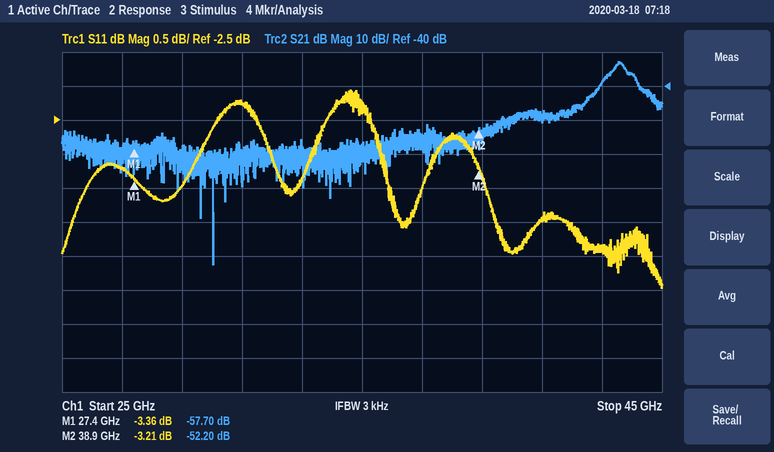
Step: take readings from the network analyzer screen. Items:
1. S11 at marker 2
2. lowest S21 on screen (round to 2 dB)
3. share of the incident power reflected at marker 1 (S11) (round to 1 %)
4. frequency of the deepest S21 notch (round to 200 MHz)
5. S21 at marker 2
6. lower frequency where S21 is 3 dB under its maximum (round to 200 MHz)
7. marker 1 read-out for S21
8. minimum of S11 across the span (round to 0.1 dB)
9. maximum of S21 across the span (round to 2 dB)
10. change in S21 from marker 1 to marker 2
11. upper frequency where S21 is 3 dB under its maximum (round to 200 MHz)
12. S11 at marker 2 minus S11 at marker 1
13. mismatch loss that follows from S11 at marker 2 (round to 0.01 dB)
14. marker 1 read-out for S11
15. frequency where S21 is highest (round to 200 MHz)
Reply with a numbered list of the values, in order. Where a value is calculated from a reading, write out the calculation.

1. -3.21 dB
2. -92 dB
3. 10^(-3.36/10) ≈ 46 %
4. 30.0 GHz
5. -52.20 dB
6. 43.4 GHz
7. -57.70 dB
8. -5.0 dB
9. -32 dB
10. -52.2 − (-57.7) = 5.50 dB
11. 43.8 GHz
12. -3.21 − (-3.36) = 0.15 dB
13. −10 log10(1 − 10^(-3.21/10)) ≈ 2.82 dB
14. -3.36 dB
15. 43.6 GHz
